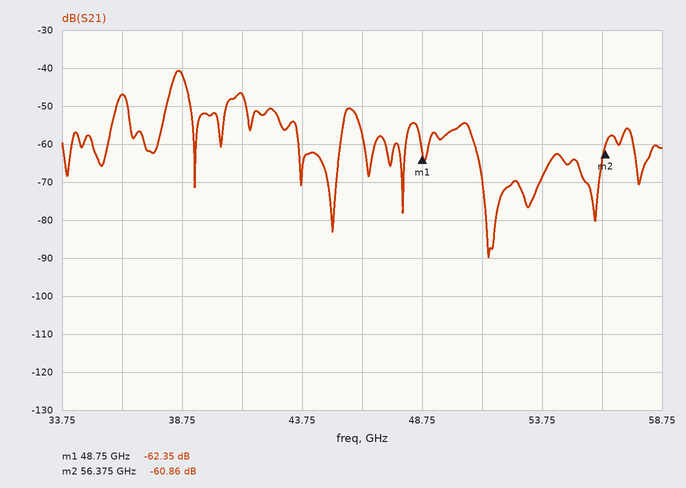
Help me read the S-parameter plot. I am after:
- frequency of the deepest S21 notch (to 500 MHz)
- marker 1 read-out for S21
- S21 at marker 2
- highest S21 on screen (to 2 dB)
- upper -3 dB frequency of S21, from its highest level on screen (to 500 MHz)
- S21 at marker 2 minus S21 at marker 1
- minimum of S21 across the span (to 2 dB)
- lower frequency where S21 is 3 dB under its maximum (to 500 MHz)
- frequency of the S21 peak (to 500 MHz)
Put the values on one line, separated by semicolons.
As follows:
51.5 GHz; -62.35 dB; -60.86 dB; -40 dB; 39.0 GHz; 1.49 dB; -90 dB; 38.5 GHz; 38.5 GHz
